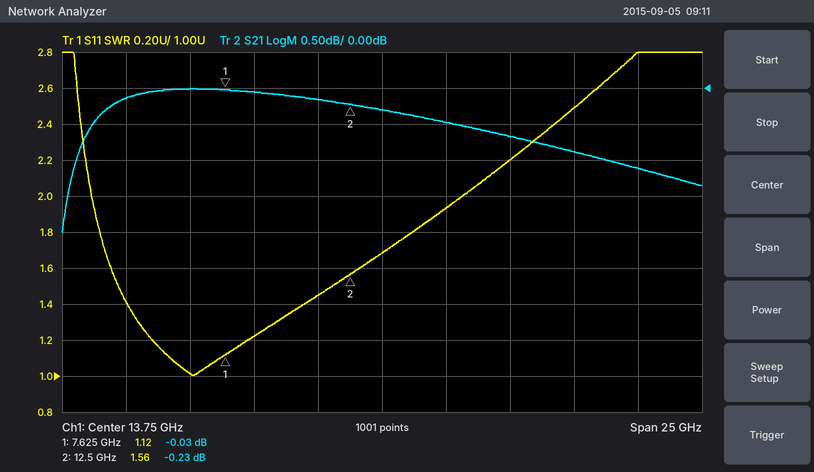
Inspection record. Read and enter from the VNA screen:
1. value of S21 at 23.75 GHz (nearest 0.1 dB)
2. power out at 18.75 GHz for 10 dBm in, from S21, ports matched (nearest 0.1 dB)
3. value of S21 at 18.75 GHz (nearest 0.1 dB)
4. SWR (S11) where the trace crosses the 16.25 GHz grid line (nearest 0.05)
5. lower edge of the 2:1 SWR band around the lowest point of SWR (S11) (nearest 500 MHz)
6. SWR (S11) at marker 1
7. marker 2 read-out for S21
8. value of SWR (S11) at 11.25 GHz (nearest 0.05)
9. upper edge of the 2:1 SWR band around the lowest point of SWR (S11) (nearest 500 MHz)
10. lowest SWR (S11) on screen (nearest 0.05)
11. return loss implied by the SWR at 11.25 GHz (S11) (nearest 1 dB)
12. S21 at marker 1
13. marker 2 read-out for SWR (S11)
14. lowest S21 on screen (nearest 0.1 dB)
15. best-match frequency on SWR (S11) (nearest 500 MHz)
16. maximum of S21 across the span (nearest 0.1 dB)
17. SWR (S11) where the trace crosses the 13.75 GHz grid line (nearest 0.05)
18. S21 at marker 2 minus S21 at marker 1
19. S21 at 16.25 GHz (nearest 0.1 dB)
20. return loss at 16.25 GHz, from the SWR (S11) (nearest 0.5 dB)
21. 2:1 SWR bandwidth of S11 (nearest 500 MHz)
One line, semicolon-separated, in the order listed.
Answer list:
-1.1 dB; 9.3 dBm; -0.7 dB; 1.95; 2.5 GHz; 1.12; -0.23 dB; 1.45; 17.0 GHz; 1.00; 15 dB; -0.03 dB; 1.56; -2.0 dB; 6.5 GHz; 0.0 dB; 1.70; -0.20 dB; -0.5 dB; 10.0 dB; 14.5 GHz
